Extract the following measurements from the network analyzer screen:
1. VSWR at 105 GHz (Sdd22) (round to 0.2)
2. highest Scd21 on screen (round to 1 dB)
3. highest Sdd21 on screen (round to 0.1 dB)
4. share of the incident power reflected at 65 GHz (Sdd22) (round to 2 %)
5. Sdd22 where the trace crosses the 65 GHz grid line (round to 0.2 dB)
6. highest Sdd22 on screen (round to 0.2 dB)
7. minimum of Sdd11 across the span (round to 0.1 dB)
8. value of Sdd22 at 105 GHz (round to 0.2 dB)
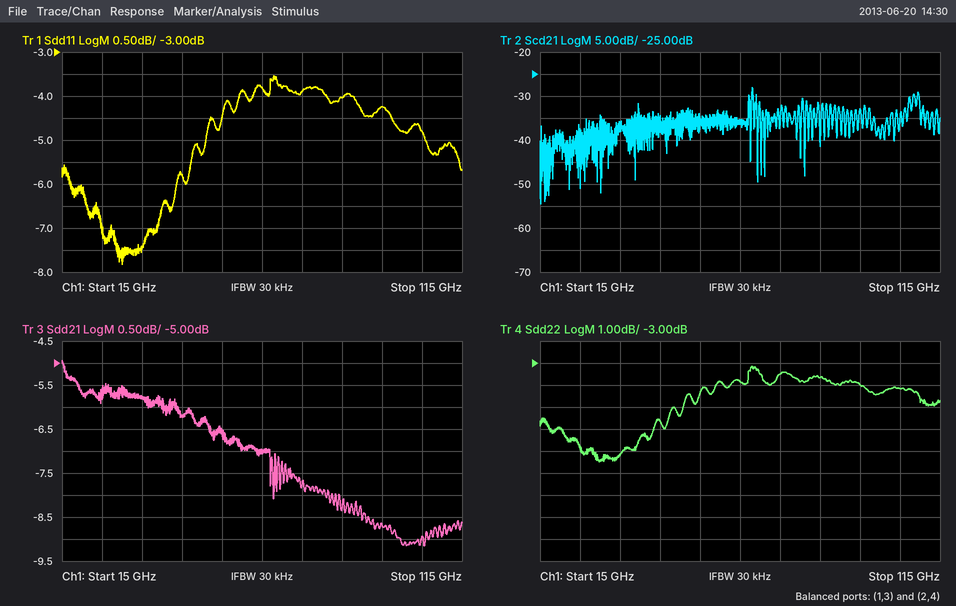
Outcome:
4.2
-28 dB
-4.9 dB
42 %
-3.8 dB
-3.2 dB
-7.8 dB
-4.2 dB
